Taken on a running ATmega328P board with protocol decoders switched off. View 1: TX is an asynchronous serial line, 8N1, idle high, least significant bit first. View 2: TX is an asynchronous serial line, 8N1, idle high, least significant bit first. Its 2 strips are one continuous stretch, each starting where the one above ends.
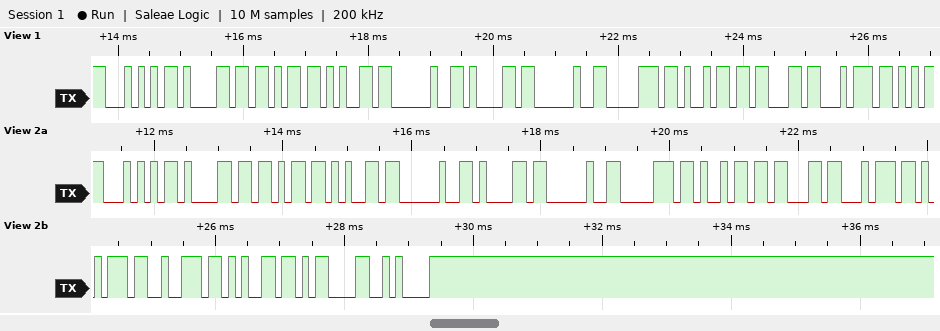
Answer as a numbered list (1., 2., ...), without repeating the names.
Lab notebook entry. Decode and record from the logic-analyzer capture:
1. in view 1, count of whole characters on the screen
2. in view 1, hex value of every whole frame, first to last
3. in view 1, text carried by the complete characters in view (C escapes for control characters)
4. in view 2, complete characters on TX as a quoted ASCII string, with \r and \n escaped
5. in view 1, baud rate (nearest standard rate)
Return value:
1. 11
2. 54 61 6B 65 20 61 20 70 69 63 74
3. "Take a pict"
4. "Take a picture\r\n"
5. 9600 baud
